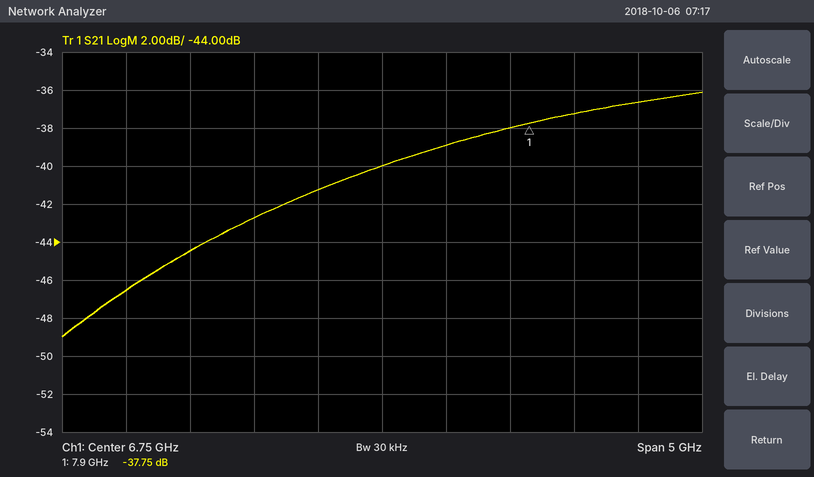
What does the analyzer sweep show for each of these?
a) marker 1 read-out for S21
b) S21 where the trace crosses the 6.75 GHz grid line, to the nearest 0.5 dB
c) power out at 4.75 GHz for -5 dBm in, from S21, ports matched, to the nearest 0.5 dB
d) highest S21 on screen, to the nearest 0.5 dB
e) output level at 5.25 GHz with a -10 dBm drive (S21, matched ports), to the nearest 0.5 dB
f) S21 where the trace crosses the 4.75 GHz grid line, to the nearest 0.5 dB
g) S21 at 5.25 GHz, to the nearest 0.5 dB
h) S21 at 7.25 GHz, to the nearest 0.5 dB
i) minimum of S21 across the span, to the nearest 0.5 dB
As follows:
-37.75 dB
-40.0 dB
-51.5 dBm
-36.0 dB
-54.5 dBm
-46.5 dB
-44.5 dB
-39.0 dB
-49.0 dB
